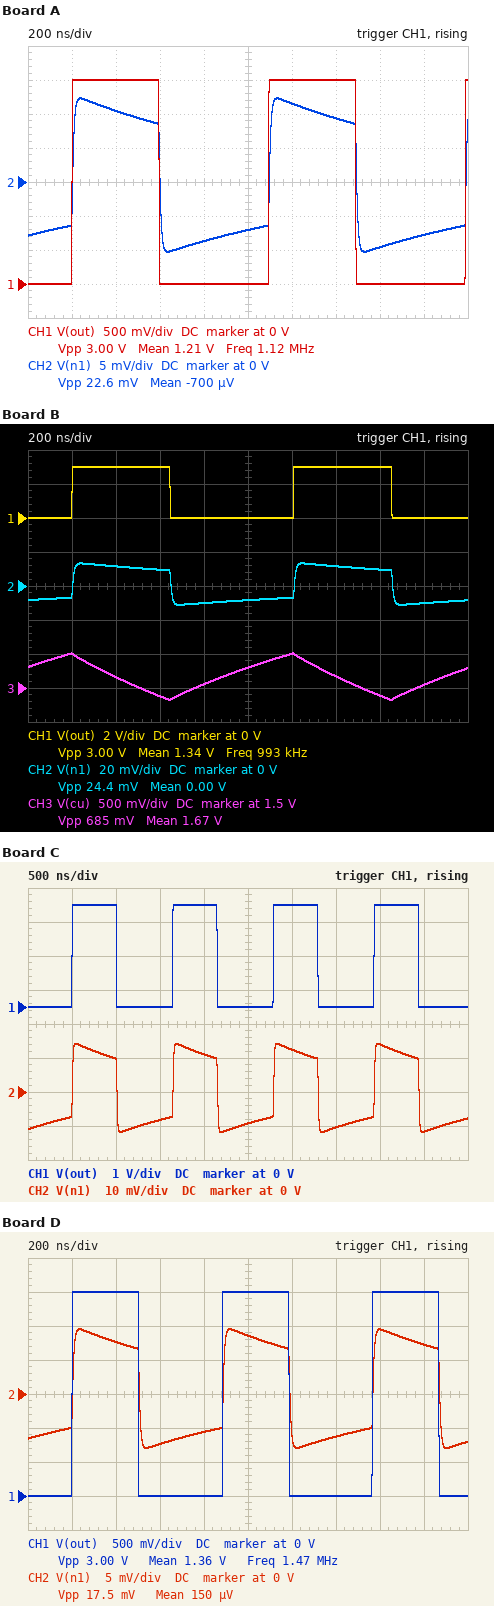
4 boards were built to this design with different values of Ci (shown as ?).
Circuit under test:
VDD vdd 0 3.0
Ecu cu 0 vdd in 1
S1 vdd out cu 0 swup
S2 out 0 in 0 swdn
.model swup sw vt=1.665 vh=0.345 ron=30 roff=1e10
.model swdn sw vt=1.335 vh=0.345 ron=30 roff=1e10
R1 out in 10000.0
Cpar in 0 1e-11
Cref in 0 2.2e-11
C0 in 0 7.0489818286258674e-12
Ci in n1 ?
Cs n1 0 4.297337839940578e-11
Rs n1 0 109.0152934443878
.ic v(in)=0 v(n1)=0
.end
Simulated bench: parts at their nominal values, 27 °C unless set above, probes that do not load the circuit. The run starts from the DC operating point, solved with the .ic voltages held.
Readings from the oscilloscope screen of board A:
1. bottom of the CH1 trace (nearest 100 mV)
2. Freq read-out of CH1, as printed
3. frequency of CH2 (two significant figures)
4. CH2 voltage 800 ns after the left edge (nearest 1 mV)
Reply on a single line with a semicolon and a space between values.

0 V; 1.12 MHz; 1.1 MHz; -9 mV
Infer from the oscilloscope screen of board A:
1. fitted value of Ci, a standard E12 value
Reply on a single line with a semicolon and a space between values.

56 pF
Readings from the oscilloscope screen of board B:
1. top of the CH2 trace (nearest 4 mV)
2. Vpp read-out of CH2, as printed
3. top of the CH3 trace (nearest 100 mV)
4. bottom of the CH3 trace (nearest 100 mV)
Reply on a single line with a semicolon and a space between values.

12 mV; 24.4 mV; 2.0 V; 1.3 V
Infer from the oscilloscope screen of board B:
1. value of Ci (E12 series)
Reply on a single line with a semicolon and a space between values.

68 pF
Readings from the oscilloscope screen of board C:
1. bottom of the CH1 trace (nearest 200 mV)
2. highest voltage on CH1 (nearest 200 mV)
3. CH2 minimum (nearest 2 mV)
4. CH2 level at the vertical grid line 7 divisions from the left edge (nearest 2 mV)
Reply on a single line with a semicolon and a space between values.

0 V; 3.0 V; -12 mV; -10 mV
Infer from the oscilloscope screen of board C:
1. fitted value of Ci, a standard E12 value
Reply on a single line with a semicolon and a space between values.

82 pF
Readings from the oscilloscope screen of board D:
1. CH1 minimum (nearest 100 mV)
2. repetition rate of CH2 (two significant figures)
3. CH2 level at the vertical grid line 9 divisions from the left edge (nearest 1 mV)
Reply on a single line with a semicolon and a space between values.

0 V; 1.5 MHz; 7 mV
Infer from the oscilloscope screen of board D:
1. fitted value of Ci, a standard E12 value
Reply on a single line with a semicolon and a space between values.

33 pF
